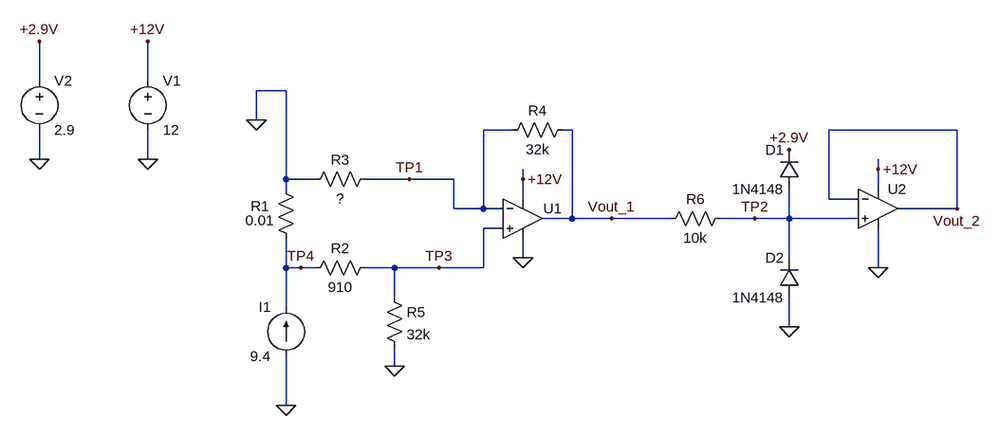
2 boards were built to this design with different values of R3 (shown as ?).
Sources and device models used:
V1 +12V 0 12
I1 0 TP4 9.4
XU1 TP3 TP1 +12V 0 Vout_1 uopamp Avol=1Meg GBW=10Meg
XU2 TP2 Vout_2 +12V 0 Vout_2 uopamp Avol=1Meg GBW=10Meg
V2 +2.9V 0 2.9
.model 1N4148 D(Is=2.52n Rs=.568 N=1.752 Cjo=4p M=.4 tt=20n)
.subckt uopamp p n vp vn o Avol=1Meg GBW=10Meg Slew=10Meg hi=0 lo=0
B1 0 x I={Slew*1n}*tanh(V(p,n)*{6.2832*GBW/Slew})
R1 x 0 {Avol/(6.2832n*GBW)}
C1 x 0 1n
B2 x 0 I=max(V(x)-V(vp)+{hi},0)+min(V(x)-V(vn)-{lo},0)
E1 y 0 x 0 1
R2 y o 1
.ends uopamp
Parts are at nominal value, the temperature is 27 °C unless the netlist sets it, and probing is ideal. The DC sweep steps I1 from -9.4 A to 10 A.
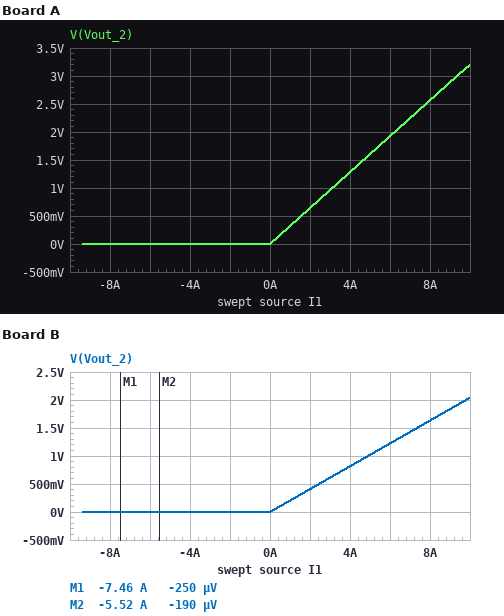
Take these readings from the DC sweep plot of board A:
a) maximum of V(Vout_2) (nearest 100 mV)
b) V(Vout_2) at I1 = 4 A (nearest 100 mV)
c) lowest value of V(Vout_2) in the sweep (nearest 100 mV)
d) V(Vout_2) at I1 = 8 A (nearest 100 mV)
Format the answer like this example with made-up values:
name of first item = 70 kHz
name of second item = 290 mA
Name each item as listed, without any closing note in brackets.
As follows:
maximum of V(Vout_2) = 3.2 V
V(Vout_2) at I1 = 4 A = 1.3 V
lowest value of V(Vout_2) in the sweep = 0 V
V(Vout_2) at I1 = 8 A = 2.6 V
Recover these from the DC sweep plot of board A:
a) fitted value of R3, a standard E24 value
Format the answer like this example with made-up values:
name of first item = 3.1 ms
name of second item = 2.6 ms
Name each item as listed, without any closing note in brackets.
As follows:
fitted value of R3, a standard E24 value = 1 kΩ
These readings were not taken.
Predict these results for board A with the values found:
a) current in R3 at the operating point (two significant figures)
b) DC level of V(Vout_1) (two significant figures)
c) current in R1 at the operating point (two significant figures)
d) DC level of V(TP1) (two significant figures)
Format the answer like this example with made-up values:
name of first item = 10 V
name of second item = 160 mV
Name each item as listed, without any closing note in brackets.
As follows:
current in R3 at the operating point = 91 µA
DC level of V(Vout_1) = 3.0 V
current in R1 at the operating point = 9.4 A
DC level of V(TP1) = 91 mV
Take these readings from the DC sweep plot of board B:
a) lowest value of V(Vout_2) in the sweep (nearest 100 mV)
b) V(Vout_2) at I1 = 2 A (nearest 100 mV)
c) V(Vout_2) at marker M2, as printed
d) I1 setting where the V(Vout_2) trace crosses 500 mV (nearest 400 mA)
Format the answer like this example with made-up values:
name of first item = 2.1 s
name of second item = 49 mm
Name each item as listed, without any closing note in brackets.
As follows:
lowest value of V(Vout_2) in the sweep = 0 V
V(Vout_2) at I1 = 2 A = 400 mV
V(Vout_2) at marker M2, as printed = -190 µV
I1 setting where the V(Vout_2) trace crosses 500 mV = 2.4 A
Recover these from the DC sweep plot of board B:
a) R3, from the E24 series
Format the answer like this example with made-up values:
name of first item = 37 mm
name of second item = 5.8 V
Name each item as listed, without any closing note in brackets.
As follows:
R3, from the E24 series = 1.6 kΩ
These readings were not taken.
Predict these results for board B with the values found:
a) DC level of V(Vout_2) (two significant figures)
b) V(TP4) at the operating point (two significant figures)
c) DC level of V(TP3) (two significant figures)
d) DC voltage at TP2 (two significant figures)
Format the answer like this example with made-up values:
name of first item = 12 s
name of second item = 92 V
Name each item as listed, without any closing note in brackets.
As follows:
DC level of V(Vout_2) = 1.9 V
V(TP4) at the operating point = 94 mV
DC level of V(TP3) = 91 mV
DC voltage at TP2 = 1.9 V
